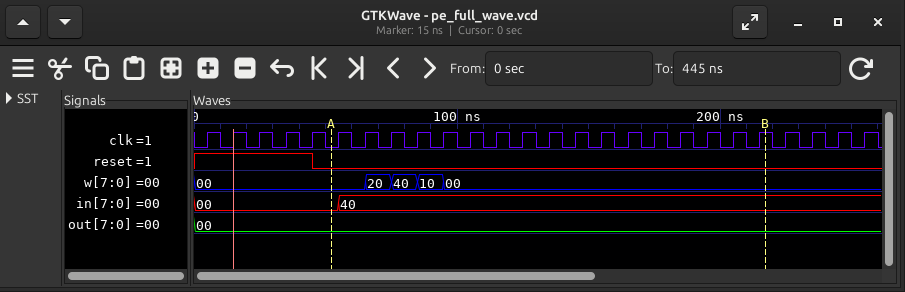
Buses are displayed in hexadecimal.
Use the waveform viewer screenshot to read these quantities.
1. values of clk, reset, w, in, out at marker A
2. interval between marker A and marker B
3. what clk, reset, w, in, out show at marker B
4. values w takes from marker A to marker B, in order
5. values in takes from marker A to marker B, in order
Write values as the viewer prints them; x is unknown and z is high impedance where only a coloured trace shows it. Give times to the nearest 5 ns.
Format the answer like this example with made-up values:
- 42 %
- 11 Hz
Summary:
- clk=0, reset=0, w=00, in=00, out=00
- 165 ns
- clk=1, reset=0, w=00, in=40, out=00
- 00, 20, 40, 10, 00
- 00, 40
